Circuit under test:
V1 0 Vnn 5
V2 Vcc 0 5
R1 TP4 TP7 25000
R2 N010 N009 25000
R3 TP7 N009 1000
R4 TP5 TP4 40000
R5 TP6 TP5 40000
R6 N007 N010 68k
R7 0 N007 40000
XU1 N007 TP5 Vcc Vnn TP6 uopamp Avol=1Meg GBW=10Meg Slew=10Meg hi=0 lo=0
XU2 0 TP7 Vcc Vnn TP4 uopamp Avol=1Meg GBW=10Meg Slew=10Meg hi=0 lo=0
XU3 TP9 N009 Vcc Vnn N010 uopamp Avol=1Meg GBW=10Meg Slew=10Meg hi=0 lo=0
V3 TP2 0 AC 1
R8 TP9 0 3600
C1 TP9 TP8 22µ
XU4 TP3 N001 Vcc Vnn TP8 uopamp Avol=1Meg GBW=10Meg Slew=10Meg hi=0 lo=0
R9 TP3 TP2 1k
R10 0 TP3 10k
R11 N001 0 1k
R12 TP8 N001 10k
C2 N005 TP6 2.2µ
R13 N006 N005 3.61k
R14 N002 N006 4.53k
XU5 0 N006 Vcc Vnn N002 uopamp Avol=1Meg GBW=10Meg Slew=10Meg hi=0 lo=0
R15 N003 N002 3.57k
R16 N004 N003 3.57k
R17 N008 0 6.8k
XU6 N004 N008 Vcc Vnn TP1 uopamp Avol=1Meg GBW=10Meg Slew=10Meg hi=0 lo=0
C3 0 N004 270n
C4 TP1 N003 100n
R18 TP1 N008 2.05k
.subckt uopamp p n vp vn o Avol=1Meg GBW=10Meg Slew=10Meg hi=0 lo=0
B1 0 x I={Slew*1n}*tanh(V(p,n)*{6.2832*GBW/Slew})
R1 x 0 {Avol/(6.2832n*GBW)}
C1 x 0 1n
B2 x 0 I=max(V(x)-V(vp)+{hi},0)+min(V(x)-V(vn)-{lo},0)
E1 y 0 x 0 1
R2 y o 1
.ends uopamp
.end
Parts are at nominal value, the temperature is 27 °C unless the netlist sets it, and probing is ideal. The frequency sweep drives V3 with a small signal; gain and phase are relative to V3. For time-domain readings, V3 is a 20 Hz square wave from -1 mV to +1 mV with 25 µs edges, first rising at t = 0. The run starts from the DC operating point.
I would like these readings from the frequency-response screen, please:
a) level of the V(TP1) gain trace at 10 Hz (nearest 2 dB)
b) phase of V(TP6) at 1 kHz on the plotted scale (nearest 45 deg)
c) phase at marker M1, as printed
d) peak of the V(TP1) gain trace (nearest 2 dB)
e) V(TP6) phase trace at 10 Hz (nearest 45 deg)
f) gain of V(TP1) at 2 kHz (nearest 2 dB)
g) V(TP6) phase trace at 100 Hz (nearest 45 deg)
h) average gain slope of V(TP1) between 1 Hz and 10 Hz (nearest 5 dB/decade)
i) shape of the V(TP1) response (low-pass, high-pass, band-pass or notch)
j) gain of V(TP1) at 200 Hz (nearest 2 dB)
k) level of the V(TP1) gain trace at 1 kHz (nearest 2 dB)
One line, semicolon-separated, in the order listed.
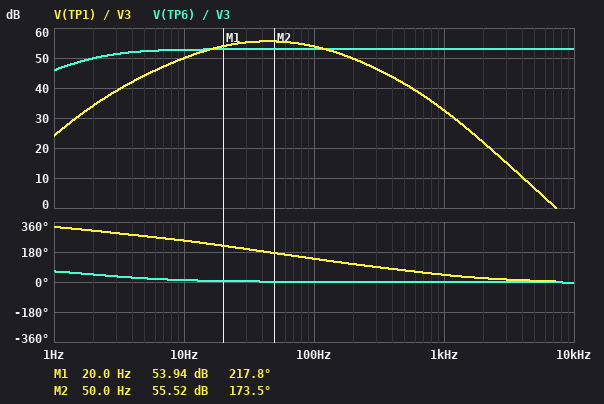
50 dB; 0 deg; 217.8 deg; 56 dB; 0 deg; 22 dB; 0 deg; 25 dB/decade; band-pass; 50 dB; 32 dB
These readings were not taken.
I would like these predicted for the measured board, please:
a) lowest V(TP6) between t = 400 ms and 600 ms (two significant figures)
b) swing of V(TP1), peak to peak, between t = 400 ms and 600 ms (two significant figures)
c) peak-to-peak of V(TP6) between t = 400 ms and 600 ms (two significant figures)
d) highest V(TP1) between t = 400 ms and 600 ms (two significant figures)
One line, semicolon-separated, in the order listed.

-510 mV; 1.9 V; 1.0 V; 950 mV
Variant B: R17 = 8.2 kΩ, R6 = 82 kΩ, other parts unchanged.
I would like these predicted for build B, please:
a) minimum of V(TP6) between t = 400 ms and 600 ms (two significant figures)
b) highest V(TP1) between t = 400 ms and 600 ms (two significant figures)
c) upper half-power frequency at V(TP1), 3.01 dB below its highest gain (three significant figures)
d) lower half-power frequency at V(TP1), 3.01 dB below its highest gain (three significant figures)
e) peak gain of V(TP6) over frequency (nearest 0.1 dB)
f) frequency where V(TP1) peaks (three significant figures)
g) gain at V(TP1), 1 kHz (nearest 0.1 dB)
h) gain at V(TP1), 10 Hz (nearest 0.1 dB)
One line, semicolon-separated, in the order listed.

-490 mV; 860 mV; 130 Hz; 14.9 Hz; 52.5 dB; 44.2 Hz; 31.7 dB; 49.2 dB
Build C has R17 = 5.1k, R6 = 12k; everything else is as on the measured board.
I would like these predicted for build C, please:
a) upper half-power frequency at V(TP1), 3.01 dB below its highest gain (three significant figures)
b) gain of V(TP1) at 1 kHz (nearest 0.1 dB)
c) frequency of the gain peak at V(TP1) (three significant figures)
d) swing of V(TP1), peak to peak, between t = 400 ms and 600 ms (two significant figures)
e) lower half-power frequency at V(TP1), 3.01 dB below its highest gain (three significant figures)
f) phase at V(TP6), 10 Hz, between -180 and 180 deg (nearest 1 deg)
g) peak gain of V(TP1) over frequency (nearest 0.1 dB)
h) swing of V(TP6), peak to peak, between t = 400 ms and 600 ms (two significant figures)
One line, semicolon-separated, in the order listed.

134 Hz; 36.6 dB; 45.0 Hz; 3.0 V; 15.1 Hz; 11 deg; 59.6 dB; 1.5 V
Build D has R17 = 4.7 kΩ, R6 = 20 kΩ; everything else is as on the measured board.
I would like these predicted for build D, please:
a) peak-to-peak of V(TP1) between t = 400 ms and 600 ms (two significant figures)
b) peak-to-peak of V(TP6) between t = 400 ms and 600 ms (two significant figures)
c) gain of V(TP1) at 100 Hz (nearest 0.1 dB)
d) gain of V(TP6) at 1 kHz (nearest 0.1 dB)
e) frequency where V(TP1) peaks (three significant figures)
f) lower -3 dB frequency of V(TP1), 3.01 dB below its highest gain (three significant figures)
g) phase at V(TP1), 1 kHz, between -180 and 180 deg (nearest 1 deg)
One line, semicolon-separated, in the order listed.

2.8 V; 1.4 V; 57.5 dB; 55.5 dB; 45.2 Hz; 15.1 Hz; 42 deg
